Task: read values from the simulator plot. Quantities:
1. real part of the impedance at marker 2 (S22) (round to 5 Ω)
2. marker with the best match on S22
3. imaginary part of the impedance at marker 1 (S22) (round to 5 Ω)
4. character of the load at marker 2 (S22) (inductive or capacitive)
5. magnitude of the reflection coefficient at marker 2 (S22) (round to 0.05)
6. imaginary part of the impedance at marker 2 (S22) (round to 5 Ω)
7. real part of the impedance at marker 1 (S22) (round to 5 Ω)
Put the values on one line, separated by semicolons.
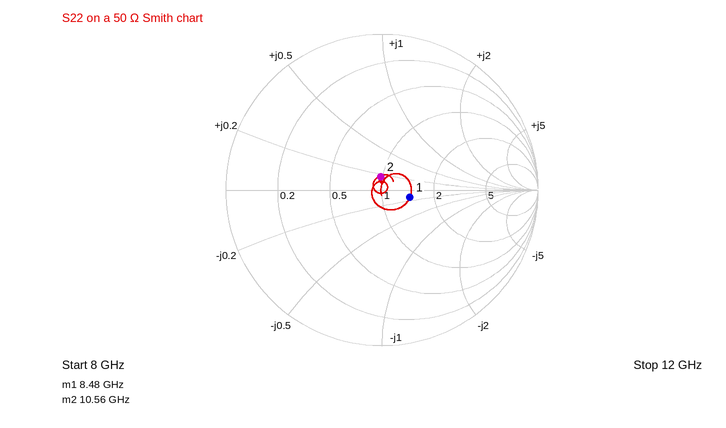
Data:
50 Ω; marker 2; -5 Ω; inductive; 0.10; +10 Ω; 70 Ω
